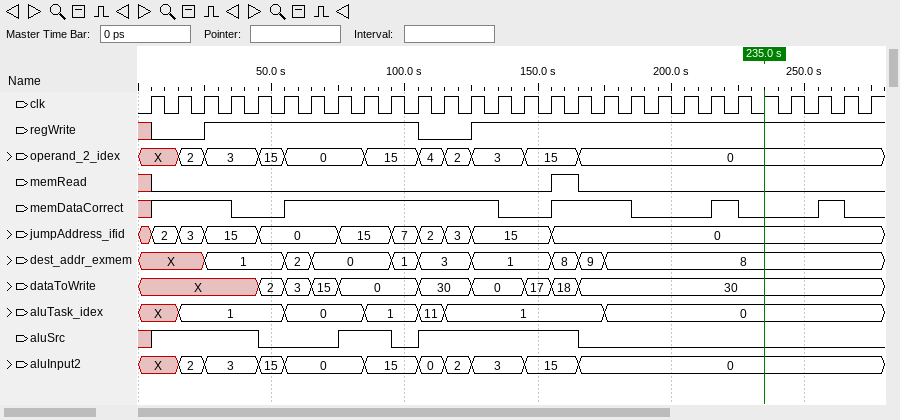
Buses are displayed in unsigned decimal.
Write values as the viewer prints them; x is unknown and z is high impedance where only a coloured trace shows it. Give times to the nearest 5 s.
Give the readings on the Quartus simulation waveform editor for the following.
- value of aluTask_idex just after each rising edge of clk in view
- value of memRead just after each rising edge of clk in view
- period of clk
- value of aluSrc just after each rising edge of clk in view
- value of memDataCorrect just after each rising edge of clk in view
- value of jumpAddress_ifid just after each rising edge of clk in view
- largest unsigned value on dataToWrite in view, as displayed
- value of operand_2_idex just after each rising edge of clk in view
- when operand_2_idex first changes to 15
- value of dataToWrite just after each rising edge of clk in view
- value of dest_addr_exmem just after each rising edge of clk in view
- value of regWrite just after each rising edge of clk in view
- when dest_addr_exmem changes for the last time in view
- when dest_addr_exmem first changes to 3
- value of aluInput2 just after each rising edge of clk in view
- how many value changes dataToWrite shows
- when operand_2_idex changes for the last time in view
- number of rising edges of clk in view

X, 1, 1, 1, 1, 0, 0, 0, 1, 1, 11, 1, 1, 1, 1, 1, 1, 0, 0, 0, 0, 0, 0, 0, 0, 0, 0, 0
0 0 0 0 0 0 0 0 0 0 0 0 0 0 0 1 0 0 0 0 0 0 0 0 0 0 0 0
10 s
1 1 1 1 0 0 0 1 1 0 1 1 1 1 1 1 0 0 0 0 0 0 0 0 0 0 0 0
1 1 1 0 0 1 1 1 1 1 1 1 1 0 0 1 1 1 0 0 0 1 0 0 0 1 0 0
2, 3, 15, 15, 0, 0, 0, 15, 15, 7, 2, 3, 15, 15, 15, 0, 0, 0, 0, 0, 0, 0, 0, 0, 0, 0, 0, 0
30
X, 2, 3, 3, 15, 0, 0, 0, 15, 15, 4, 2, 3, 3, 15, 15, 0, 0, 0, 0, 0, 0, 0, 0, 0, 0, 0, 0
45 s
X, X, X, X, 2, 3, 15, 0, 0, 0, 30, 30, 0, 0, 17, 18, 30, 30, 30, 30, 30, 30, 30, 30, 30, 30, 30, 30
X, X, 1, 1, 1, 2, 0, 0, 0, 1, 3, 3, 1, 1, 1, 8, 9, 8, 8, 8, 8, 8, 8, 8, 8, 8, 8, 8
0 0 1 1 1 1 1 1 1 1 0 0 1 1 1 1 1 1 1 1 1 1 1 1 1 1 1 1
175 s
105 s
X, 2, 3, 3, 15, 0, 0, 0, 15, 15, 0, 2, 3, 3, 15, 15, 0, 0, 0, 0, 0, 0, 0, 0, 0, 0, 0, 0
9
165 s
28
